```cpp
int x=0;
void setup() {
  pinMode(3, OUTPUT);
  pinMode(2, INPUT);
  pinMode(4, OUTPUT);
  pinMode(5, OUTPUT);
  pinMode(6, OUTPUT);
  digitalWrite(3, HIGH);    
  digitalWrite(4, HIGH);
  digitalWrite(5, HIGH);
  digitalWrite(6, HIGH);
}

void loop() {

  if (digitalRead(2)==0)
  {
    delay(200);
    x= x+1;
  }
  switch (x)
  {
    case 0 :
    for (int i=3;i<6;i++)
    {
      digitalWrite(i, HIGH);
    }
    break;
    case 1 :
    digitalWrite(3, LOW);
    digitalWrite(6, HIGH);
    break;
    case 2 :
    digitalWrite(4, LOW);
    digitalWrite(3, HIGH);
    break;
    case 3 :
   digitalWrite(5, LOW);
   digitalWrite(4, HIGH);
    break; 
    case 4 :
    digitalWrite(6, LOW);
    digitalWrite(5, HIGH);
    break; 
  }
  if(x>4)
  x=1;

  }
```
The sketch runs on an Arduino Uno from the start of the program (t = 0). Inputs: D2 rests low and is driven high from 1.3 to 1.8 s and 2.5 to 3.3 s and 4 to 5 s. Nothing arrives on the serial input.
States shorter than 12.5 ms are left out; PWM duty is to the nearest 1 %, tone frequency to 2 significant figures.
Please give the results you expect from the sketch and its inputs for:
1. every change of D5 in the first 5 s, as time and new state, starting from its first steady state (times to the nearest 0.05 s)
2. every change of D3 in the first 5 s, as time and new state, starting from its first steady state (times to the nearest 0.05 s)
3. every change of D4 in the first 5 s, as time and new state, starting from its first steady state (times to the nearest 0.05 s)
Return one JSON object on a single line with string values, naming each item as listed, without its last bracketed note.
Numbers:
{"every change of D5 in the first 5 s, as time and new state, starting from its first steady state": "0 s high; 0.6 s low; 0.8 s high; 1.4 s low; 2 s high; 2.6 s low; 3.5 s high; 4.1 s low", "every change of D3 in the first 5 s, as time and new state, starting from its first steady state": "0 s high; 0.2 s low; 0.4 s high", "every change of D4 in the first 5 s, as time and new state, starting from its first steady state": "0 s high; 0.4 s low; 0.6 s high; 1.2 s low; 1.4 s high; 2.4 s low; 2.6 s high; 3.9 s low; 4.1 s high"}
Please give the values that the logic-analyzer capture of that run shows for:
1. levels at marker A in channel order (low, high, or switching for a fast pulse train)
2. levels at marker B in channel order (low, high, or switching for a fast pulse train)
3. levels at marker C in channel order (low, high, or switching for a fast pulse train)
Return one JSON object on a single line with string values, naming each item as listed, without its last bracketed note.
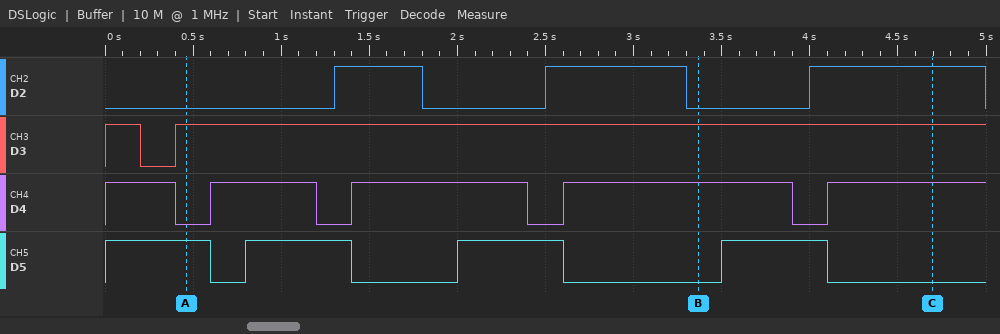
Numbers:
{"levels at marker A in channel order": "D2 low, D3 high, D4 low, D5 high", "levels at marker B in channel order": "D2 low, D3 high, D4 high, D5 low", "levels at marker C in channel order": "D2 high, D3 high, D4 high, D5 low"}
